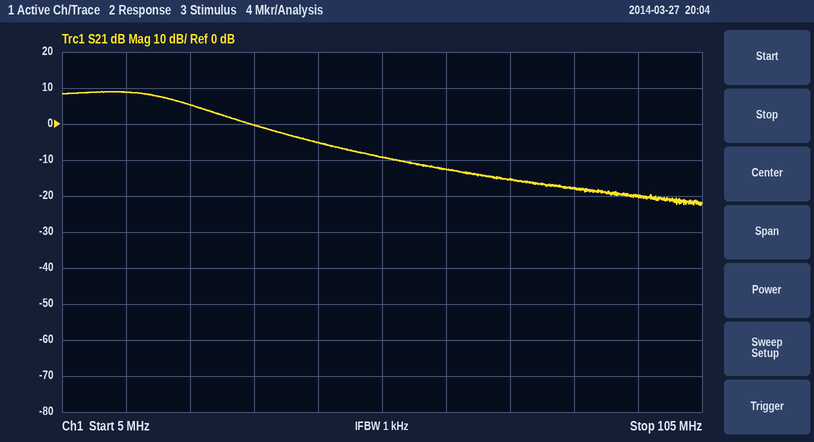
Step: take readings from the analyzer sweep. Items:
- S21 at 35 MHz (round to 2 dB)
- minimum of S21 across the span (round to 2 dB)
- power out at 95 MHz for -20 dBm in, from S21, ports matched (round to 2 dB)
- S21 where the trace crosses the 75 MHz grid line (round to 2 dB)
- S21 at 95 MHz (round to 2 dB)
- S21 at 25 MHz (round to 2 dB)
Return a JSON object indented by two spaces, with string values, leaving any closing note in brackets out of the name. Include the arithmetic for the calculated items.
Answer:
{
  "S21 at 35 MHz": "0 dB",
  "minimum of S21 across the span": "-22 dB",
  "power out at 95 MHz for -20 dBm in, from S21, ports matched": "-20 dBm + (-20 dB) = -40 dBm",
  "S21 where the trace crosses the 75 MHz grid line": "-16 dB",
  "S21 at 95 MHz": "-20 dB",
  "S21 at 25 MHz": "6 dB"
}
